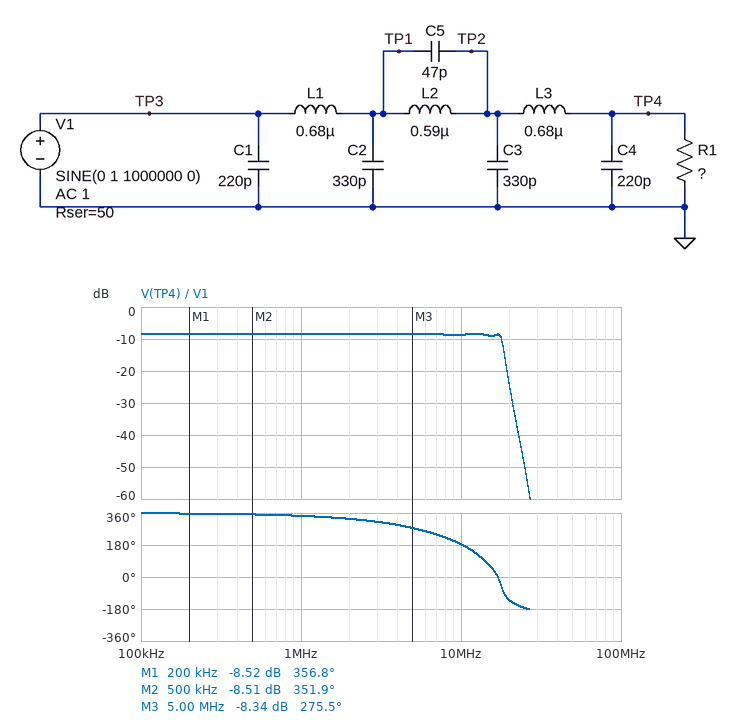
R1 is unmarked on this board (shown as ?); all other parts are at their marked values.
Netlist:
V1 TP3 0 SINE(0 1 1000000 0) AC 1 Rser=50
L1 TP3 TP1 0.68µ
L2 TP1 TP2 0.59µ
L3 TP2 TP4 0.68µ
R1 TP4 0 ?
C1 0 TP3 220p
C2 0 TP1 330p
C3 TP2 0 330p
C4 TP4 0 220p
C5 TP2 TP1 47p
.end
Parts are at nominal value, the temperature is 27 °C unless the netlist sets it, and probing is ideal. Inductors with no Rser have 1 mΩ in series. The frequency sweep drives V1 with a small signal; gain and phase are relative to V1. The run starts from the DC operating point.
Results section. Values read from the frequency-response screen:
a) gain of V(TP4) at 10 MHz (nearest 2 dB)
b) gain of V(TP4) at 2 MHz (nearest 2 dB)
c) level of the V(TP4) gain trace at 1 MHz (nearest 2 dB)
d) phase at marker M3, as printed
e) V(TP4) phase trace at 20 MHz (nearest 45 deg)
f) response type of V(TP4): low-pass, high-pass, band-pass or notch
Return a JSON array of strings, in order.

["-8 dB", "-8 dB", "-8 dB", "275.5 deg", "-135 deg", "low-pass"]
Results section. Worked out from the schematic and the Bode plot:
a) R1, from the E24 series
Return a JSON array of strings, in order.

["30 Ω"]
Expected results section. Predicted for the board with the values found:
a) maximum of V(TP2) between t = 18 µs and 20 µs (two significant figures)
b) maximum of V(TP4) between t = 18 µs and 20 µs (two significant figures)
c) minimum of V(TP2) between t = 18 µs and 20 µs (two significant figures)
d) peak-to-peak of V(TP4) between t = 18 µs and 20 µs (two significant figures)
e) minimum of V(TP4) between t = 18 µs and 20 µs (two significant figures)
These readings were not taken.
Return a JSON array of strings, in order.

["380 mV", "380 mV", "-380 mV", "750 mV", "-380 mV"]
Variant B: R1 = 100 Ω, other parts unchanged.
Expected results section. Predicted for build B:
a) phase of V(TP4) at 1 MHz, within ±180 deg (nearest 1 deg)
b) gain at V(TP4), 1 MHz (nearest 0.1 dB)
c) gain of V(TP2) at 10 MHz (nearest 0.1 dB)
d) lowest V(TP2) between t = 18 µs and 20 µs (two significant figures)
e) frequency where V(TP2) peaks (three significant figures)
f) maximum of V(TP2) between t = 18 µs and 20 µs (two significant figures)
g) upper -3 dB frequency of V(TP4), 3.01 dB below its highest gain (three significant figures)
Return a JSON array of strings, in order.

["-18 deg", "-3.6 dB", "-8.2 dB", "-660 mV", "18.1 MHz", "660 mV", "18.8 MHz"]
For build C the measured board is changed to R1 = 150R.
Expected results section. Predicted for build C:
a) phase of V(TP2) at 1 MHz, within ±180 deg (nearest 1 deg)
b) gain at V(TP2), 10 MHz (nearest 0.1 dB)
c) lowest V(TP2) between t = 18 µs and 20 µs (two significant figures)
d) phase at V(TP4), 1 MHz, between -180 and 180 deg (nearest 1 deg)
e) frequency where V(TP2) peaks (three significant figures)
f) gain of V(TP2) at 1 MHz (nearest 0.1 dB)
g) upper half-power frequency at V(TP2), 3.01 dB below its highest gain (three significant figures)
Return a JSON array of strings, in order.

["-17 deg", "-8.7 dB", "-740 mV", "-18 deg", "18.4 MHz", "-2.6 dB", "19.1 MHz"]
